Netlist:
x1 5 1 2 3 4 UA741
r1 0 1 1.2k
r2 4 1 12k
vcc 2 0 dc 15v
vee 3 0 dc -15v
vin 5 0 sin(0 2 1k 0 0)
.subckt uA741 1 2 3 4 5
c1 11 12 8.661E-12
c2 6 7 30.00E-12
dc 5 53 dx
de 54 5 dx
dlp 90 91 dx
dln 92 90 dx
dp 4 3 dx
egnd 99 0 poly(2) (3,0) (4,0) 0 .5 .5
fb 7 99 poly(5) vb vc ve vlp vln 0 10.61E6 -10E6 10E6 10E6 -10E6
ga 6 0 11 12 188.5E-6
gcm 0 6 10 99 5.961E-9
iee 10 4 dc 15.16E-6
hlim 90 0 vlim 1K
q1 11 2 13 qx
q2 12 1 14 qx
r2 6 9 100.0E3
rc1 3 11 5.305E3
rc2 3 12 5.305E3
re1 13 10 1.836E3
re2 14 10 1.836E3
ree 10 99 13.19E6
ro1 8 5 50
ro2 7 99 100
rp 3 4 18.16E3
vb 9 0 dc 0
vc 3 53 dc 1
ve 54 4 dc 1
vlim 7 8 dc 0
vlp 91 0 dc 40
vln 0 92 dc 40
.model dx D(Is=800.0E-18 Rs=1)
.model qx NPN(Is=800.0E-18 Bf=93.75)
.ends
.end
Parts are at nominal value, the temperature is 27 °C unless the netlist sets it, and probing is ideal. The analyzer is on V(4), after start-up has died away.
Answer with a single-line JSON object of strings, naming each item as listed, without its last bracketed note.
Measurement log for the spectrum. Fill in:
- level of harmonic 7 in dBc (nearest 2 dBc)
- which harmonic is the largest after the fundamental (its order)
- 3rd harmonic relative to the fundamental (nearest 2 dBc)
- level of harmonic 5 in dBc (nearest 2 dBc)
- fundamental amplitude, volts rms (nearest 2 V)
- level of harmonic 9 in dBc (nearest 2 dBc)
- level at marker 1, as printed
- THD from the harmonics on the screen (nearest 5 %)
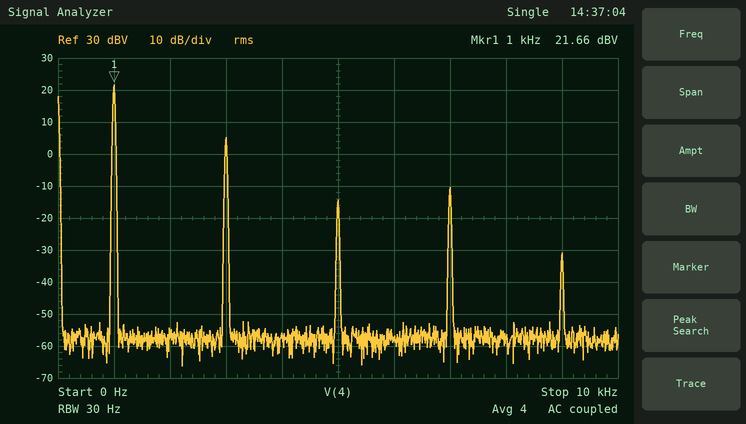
{"level of harmonic 7 in dBc": "-32 dBc", "which harmonic is the largest after the fundamental": "3", "3rd harmonic relative to the fundamental": "-16 dBc", "level of harmonic 5 in dBc": "-36 dBc", "fundamental amplitude, volts rms": "12 V", "level of harmonic 9 in dBc": "-52 dBc", "level at marker 1, as printed": "21.66 dBV", "THD from the harmonics on the screen": "15 %"}
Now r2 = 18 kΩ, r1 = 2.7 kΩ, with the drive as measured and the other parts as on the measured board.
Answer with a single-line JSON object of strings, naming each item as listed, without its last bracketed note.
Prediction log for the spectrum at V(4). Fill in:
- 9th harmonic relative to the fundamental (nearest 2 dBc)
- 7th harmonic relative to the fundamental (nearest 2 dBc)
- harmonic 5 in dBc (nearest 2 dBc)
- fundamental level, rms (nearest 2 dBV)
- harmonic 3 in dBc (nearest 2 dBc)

{"9th harmonic relative to the fundamental": "-46 dBc", "7th harmonic relative to the fundamental": "-42 dBc", "harmonic 5 in dBc": "-40 dBc", "fundamental level, rms": "20 dBV", "harmonic 3 in dBc": "-38 dBc"}
